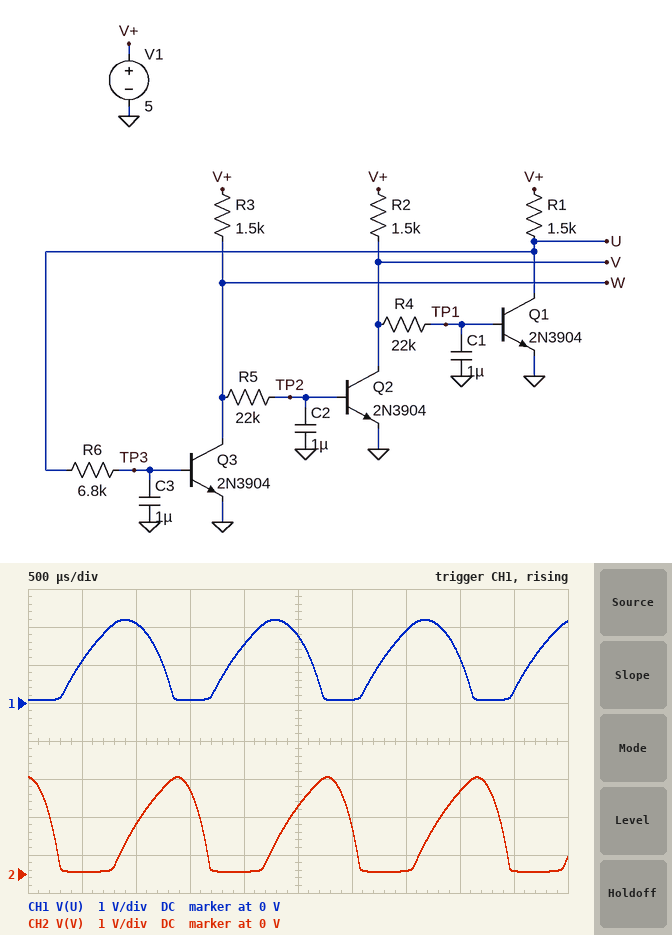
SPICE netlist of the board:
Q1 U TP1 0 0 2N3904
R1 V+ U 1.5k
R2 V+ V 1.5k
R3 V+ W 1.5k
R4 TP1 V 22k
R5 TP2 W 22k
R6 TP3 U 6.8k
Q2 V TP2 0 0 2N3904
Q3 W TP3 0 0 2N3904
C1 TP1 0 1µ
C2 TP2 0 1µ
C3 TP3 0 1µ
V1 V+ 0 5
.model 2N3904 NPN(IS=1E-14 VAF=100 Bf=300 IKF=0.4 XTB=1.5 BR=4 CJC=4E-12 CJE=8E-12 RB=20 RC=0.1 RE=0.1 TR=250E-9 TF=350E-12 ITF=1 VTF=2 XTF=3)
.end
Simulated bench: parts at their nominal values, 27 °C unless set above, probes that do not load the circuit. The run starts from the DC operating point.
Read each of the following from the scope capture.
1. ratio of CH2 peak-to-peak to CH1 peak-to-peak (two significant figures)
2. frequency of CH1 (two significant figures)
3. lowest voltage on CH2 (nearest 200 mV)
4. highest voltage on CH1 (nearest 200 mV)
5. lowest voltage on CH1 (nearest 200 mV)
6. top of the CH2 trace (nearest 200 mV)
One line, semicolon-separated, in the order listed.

1.2; 720 Hz; 0 V; 2.2 V; 0 V; 2.6 V
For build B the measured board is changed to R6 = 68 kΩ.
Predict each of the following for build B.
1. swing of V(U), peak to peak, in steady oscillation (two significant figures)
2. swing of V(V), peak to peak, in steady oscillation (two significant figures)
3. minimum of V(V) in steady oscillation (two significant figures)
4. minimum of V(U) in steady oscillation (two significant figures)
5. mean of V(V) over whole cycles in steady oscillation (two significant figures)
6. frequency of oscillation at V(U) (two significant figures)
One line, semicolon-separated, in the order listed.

3.4 V; 2.9 V; 72 mV; 62 mV; 1.3 V; 390 Hz
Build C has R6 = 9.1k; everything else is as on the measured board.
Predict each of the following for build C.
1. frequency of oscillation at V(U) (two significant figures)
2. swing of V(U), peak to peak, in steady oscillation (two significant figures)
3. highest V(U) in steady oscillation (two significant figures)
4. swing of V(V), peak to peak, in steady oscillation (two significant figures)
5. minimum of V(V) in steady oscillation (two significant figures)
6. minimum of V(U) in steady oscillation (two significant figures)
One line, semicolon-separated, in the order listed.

690 Hz; 2.2 V; 2.3 V; 2.5 V; 60 mV; 70 mV
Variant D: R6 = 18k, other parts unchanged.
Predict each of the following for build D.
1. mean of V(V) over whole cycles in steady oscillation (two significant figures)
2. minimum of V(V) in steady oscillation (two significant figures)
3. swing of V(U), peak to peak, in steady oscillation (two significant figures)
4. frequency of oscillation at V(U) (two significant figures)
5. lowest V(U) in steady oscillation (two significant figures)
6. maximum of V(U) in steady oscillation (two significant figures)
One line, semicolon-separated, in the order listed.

1.2 V; 65 mV; 2.5 V; 590 Hz; 67 mV; 2.6 V
